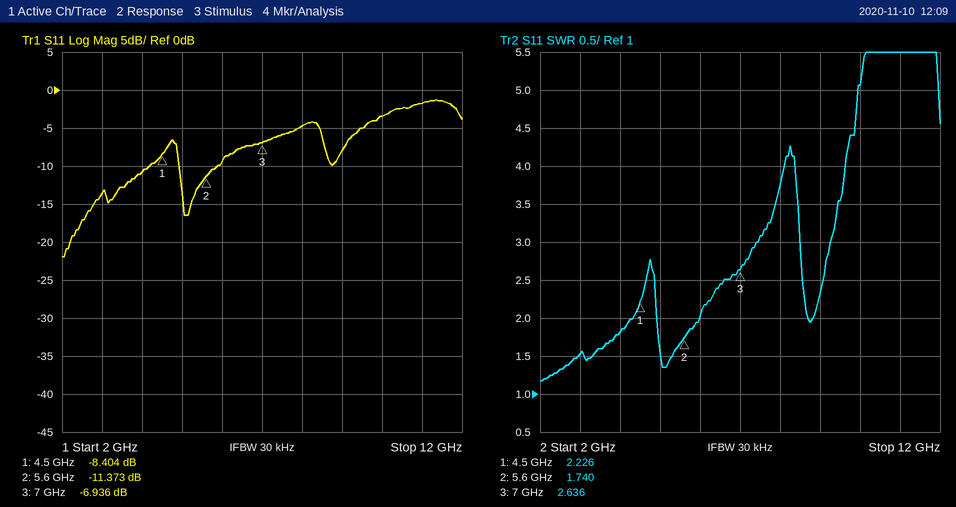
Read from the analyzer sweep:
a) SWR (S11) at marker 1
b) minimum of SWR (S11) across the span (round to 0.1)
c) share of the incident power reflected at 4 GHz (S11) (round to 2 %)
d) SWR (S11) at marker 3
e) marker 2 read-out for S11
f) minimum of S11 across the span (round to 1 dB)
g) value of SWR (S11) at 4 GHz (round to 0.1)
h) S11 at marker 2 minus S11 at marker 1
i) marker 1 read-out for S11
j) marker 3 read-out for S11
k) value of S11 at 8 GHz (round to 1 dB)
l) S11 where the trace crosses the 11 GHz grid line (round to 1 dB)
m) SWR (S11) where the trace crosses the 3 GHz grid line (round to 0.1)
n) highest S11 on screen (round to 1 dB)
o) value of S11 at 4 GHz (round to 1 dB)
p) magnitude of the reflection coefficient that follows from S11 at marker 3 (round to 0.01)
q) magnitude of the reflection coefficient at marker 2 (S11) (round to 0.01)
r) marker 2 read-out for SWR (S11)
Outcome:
2.226
1.2
8 %
2.636
-11.373 dB
-22 dB
1.8
-2.969 dB
-8.404 dB
-6.936 dB
-5 dB
-2 dB
1.5
-1 dB
-11 dB
0.45
0.27
1.740
